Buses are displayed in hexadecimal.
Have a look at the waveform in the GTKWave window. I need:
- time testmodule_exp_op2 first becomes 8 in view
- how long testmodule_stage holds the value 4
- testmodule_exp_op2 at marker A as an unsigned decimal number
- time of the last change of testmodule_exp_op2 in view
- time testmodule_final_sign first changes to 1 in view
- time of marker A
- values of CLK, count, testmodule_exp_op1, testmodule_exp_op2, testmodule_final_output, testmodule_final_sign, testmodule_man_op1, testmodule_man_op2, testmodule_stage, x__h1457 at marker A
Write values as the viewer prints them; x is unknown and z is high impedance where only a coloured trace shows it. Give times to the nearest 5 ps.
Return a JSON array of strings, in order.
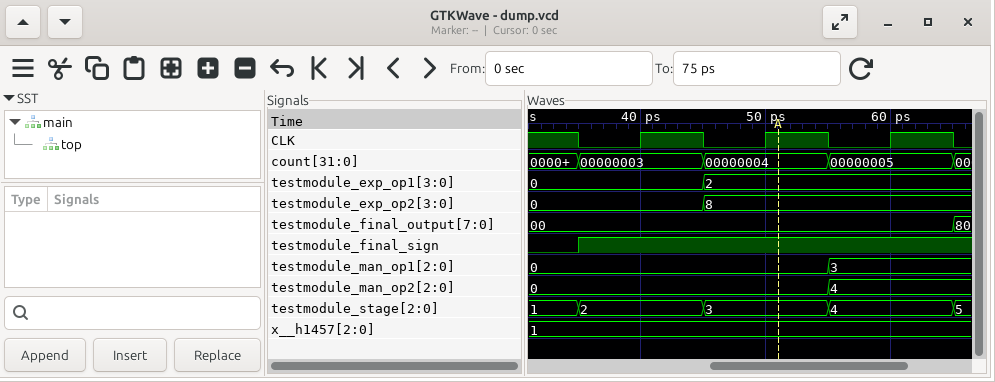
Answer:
["45 ps", "10 ps", "8", "45 ps", "35 ps", "50 ps", "CLK=1, count=00000004, testmodule_exp_op1=2, testmodule_exp_op2=8, testmodule_final_output=00, testmodule_final_sign=1, testmodule_man_op1=0, testmodule_man_op2=0, testmodule_stage=3, x__h1457=1"]
